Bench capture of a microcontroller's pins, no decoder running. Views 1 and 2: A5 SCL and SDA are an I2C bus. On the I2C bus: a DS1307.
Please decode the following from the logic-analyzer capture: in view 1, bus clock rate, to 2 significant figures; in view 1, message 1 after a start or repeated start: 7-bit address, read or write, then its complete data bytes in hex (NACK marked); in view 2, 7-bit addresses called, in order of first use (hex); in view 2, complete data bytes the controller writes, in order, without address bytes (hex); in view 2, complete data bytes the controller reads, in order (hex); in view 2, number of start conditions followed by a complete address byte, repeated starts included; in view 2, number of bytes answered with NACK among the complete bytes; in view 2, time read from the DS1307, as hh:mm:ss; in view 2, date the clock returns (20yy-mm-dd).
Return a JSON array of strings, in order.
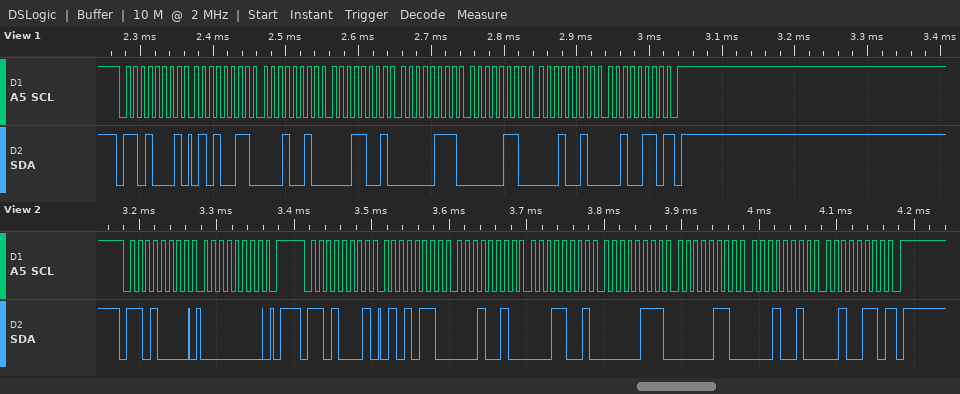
["100 kHz", "0x68 read: 53 12 19 07 06 12 26 NACK", "0x68", "00", "56 12 19 07 06 12 26", "2", "1", "19:12:56", "2026-12-06"]
